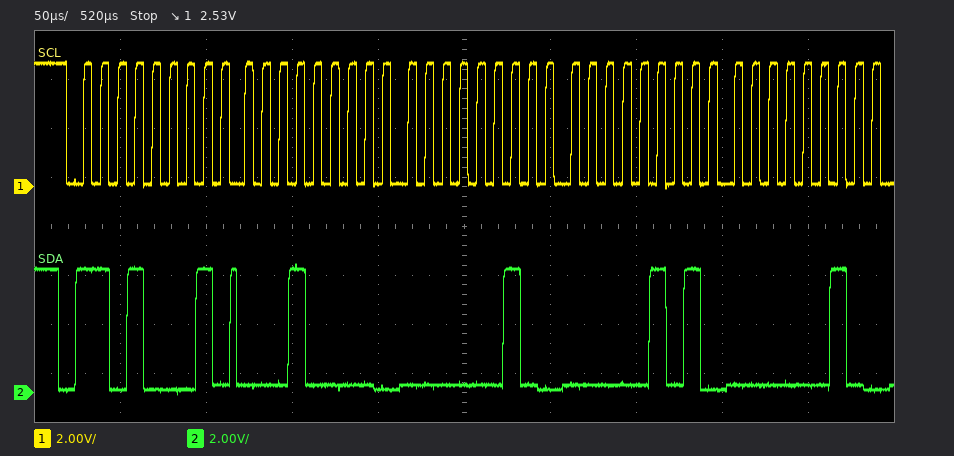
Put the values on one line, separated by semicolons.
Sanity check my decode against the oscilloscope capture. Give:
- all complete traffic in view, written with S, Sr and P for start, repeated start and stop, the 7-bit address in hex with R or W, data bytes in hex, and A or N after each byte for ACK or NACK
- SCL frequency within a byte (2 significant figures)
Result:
S 68R A 10 A 02 A 05 A 02 A; 100 kHz
